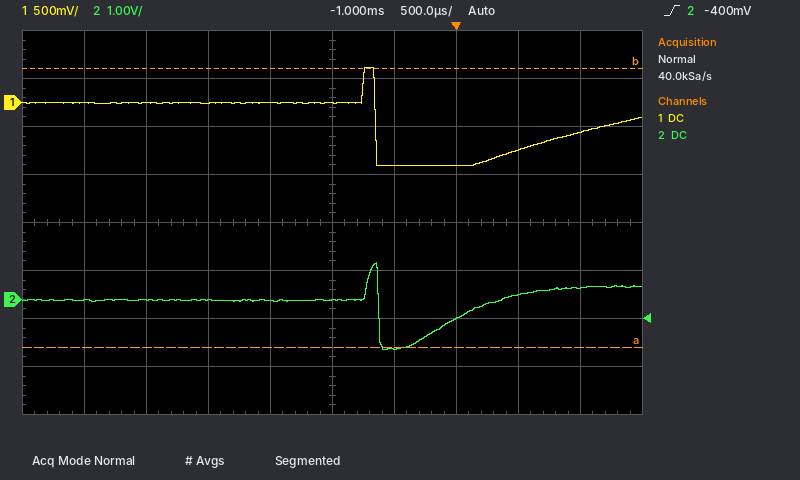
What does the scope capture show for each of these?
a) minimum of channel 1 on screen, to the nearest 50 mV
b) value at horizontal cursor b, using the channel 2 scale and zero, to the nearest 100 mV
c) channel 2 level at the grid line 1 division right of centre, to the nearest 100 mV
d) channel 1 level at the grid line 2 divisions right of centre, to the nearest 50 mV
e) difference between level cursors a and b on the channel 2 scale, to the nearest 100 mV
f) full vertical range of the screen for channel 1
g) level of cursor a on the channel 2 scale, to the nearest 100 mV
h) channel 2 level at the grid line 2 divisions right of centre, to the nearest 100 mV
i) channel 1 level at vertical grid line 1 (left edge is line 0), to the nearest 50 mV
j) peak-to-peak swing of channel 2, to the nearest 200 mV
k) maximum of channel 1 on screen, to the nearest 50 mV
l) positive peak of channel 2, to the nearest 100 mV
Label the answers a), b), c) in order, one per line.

a) -650 mV
b) 4.8 V
c) -1.0 V
d) -650 mV
e) 5.8 V
f) 4 V
g) -1.0 V
h) -400 mV
i) 0 mV
j) 1.8 V
k) 350 mV
l) 800 mV
